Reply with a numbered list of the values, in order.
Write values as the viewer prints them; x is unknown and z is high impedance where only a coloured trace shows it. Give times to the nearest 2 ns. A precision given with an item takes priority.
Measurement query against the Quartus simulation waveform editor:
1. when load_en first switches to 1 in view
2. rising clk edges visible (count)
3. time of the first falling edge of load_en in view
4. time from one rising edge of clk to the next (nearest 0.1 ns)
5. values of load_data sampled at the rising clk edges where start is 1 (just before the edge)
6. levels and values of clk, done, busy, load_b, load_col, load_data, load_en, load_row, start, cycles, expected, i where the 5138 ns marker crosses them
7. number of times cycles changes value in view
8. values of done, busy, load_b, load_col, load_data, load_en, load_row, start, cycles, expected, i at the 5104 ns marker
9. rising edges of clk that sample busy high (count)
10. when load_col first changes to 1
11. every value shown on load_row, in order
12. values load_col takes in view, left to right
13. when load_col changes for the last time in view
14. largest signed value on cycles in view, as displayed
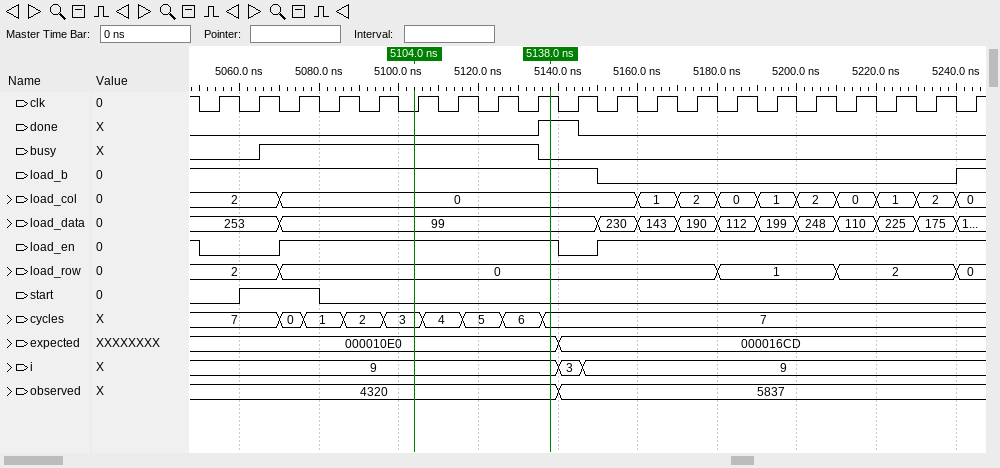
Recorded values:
1. 5070 ns
2. 20
3. 5050 ns
4. 10 ns
5. 253, 99
6. clk=1, done=1, busy=0, load_b=1, load_col=0, load_data=99, load_en=1, load_row=0, start=0, cycles=7, expected=000010E0, i=9
7. 8
8. done=0, busy=1, load_b=1, load_col=0, load_data=99, load_en=1, load_row=0, start=0, cycles=3, expected=000010E0, i=9
9. 7
10. 5160 ns
11. 2, 0, 1, 2, 0
12. 2, 0, 1, 2, 0, 1, 2, 0, 1, 2, 0
13. 5240 ns
14. 7
